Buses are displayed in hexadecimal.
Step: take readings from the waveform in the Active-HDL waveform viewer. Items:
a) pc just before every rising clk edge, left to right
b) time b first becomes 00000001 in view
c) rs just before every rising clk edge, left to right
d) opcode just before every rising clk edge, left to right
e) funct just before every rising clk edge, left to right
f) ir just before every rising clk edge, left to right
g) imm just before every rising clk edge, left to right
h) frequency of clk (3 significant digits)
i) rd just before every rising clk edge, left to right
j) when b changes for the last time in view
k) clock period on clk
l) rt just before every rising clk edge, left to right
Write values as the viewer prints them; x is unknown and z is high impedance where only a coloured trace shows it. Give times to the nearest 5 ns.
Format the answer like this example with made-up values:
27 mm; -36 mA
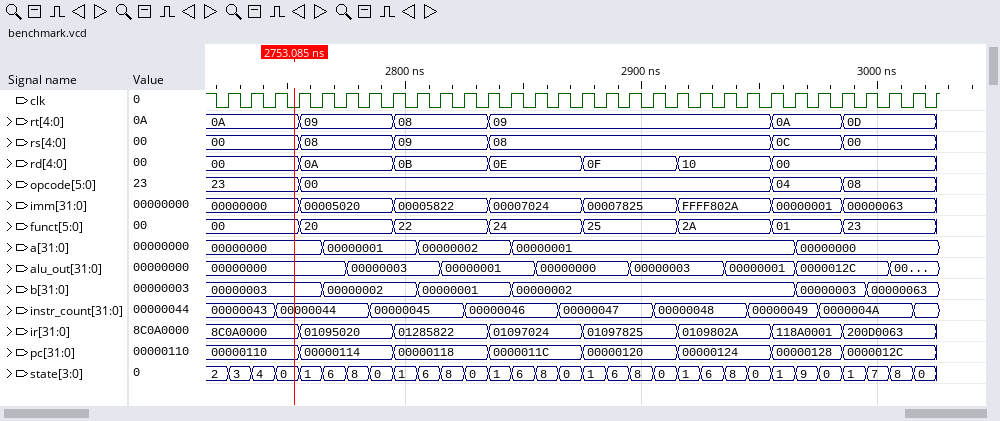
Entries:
00000110, 00000110, 00000110, 00000110, 00000114, 00000114, 00000114, 00000114, 00000118, 00000118, 00000118, 00000118, 0000011C, 0000011C, 0000011C, 0000011C, 00000120, 00000120, 00000120, 00000120, 00000124, 00000124, 00000124, 00000124, 00000128, 00000128, 00000128, 0000012C, 0000012C, 0000012C, 0000012C; 2805 ns; 00, 00, 00, 00, 08, 08, 08, 08, 09, 09, 09, 09, 08, 08, 08, 08, 08, 08, 08, 08, 08, 08, 08, 08, 0C, 0C, 0C, 00, 00, 00, 00; 23, 23, 23, 23, 00, 00, 00, 00, 00, 00, 00, 00, 00, 00, 00, 00, 00, 00, 00, 00, 00, 00, 00, 00, 04, 04, 04, 08, 08, 08, 08; 00, 00, 00, 00, 20, 20, 20, 20, 22, 22, 22, 22, 24, 24, 24, 24, 25, 25, 25, 25, 2A, 2A, 2A, 2A, 01, 01, 01, 23, 23, 23, 23; 8C0A0000, 8C0A0000, 8C0A0000, 8C0A0000, 01095020, 01095020, 01095020, 01095020, 01285822, 01285822, 01285822, 01285822, 01097024, 01097024, 01097024, 01097024, 01097825, 01097825, 01097825, 01097825, 0109802A, 0109802A, 0109802A, 0109802A, 118A0001, 118A0001, 118A0001, 200D0063, 200D0063, 200D0063, 200D0063; 00000000, 00000000, 00000000, 00000000, 00005020, 00005020, 00005020, 00005020, 00005822, 00005822, 00005822, 00005822, 00007024, 00007024, 00007024, 00007024, 00007825, 00007825, 00007825, 00007825, FFFF802A, FFFF802A, FFFF802A, FFFF802A, 00000001, 00000001, 00000001, 00000063, 00000063, 00000063, 00000063; 100 MHz; 00, 00, 00, 00, 0A, 0A, 0A, 0A, 0B, 0B, 0B, 0B, 0E, 0E, 0E, 0E, 0F, 0F, 0F, 0F, 10, 10, 10, 10, 00, 00, 00, 00, 00, 00, 00; 2995 ns; 10 ns; 0A, 0A, 0A, 0A, 09, 09, 09, 09, 08, 08, 08, 08, 09, 09, 09, 09, 09, 09, 09, 09, 09, 09, 09, 09, 0A, 0A, 0A, 0D, 0D, 0D, 0D
